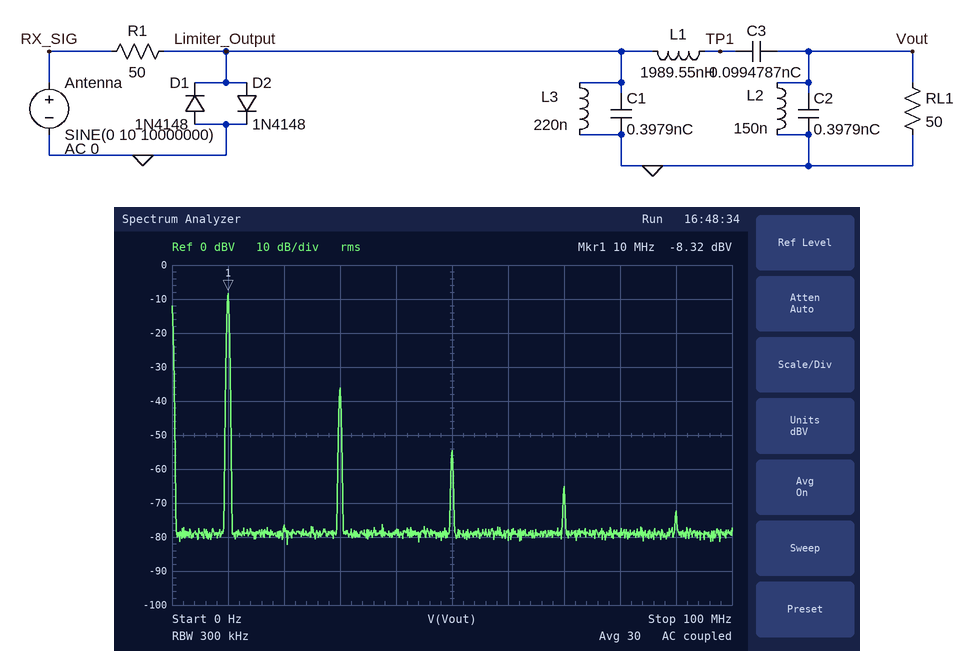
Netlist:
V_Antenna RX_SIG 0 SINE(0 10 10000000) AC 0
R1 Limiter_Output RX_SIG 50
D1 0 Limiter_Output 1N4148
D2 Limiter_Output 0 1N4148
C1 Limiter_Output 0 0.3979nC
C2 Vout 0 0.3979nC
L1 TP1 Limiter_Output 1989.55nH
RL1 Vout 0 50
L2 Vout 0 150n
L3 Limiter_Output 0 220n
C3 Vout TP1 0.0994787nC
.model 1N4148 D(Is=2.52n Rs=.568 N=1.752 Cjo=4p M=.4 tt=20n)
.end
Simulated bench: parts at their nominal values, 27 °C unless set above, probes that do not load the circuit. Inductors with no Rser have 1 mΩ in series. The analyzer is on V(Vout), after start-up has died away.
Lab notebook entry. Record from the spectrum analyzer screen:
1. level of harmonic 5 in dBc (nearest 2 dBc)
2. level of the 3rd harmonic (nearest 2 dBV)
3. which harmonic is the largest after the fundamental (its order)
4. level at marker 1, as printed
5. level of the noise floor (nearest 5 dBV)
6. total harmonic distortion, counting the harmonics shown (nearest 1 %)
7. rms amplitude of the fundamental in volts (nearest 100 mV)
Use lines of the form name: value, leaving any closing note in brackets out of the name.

level of harmonic 5 in dBc: -46 dBc
level of the 3rd harmonic: -36 dBV
which harmonic is the largest after the fundamental: 3
level at marker 1, as printed: -8.32 dBV
level of the noise floor: -80 dBV
total harmonic distortion, counting the harmonics shown: 4 %
rms amplitude of the fundamental in volts: 400 mV
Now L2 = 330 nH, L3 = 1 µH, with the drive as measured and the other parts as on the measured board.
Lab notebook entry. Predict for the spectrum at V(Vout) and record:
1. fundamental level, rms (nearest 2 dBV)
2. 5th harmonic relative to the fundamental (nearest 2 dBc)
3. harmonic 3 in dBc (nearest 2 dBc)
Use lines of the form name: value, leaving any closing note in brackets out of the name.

fundamental level, rms: 0 dBV
5th harmonic relative to the fundamental: -56 dBc
harmonic 3 in dBc: -40 dBc
